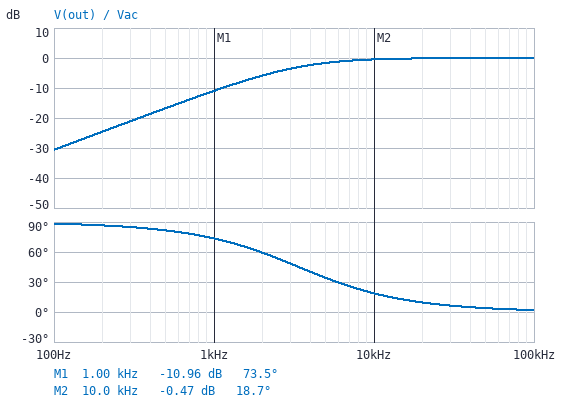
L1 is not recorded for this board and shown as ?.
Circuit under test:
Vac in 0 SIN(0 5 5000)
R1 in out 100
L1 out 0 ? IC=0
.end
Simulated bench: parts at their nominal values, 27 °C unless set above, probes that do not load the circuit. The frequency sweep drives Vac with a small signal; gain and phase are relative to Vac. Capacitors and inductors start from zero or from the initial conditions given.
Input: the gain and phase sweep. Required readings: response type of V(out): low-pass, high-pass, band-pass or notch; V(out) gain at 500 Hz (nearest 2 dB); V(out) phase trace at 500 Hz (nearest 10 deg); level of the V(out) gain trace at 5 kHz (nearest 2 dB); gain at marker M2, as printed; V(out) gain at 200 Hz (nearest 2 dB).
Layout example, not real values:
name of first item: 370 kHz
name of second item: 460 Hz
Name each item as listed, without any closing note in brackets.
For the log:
response type of V(out): low-pass, high-pass, band-pass or notch: high-pass
V(out) gain at 500 Hz: -16 dB
V(out) phase trace at 500 Hz: 80 deg
level of the V(out) gain trace at 5 kHz: -2 dB
gain at marker M2, as printed: -0.47 dB
V(out) gain at 200 Hz: -24 dB
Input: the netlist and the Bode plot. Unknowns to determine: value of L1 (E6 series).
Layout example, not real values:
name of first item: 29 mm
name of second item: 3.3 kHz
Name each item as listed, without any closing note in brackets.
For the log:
value of L1: 4.7 mH
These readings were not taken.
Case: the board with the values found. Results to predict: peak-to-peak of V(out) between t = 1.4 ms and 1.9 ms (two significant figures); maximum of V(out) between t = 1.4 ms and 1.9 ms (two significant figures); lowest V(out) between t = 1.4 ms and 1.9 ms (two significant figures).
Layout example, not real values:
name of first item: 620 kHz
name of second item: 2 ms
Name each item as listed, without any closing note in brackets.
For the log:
peak-to-peak of V(out) between t = 1.4 ms and 1.9 ms: 8.3 V
maximum of V(out) between t = 1.4 ms and 1.9 ms: 4.1 V
lowest V(out) between t = 1.4 ms and 1.9 ms: -4.1 V
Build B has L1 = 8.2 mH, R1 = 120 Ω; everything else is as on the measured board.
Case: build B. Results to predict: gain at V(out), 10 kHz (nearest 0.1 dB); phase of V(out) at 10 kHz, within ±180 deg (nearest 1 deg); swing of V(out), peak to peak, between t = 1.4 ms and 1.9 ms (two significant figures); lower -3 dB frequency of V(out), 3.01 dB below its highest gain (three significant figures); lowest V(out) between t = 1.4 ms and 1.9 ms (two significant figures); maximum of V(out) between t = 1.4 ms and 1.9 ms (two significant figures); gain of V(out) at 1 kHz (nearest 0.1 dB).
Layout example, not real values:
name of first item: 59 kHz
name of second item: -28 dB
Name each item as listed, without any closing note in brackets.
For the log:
gain at V(out), 10 kHz: -0.2 dB
phase of V(out) at 10 kHz, within ±180 deg: 13 deg
swing of V(out), peak to peak, between t = 1.4 ms and 1.9 ms: 9.1 V
lower -3 dB frequency of V(out), 3.01 dB below its highest gain: 2.33 kHz
lowest V(out) between t = 1.4 ms and 1.9 ms: -4.5 V
maximum of V(out) between t = 1.4 ms and 1.9 ms: 4.5 V
gain of V(out) at 1 kHz: -8.1 dB
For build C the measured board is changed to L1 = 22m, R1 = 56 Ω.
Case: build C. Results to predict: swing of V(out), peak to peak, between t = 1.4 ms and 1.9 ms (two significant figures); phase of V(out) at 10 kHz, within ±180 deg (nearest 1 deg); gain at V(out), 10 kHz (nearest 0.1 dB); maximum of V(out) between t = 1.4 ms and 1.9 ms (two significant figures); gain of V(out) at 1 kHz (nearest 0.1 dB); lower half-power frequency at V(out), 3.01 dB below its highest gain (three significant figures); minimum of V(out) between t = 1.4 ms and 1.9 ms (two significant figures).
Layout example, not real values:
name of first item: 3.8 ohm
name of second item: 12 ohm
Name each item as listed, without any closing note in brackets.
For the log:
swing of V(out), peak to peak, between t = 1.4 ms and 1.9 ms: 10 V
phase of V(out) at 10 kHz, within ±180 deg: 2 deg
gain at V(out), 10 kHz: 0 dB
maximum of V(out) between t = 1.4 ms and 1.9 ms: 5.0 V
gain of V(out) at 1 kHz: -0.7 dB
lower half-power frequency at V(out), 3.01 dB below its highest gain: 405 Hz
minimum of V(out) between t = 1.4 ms and 1.9 ms: -5.0 V
